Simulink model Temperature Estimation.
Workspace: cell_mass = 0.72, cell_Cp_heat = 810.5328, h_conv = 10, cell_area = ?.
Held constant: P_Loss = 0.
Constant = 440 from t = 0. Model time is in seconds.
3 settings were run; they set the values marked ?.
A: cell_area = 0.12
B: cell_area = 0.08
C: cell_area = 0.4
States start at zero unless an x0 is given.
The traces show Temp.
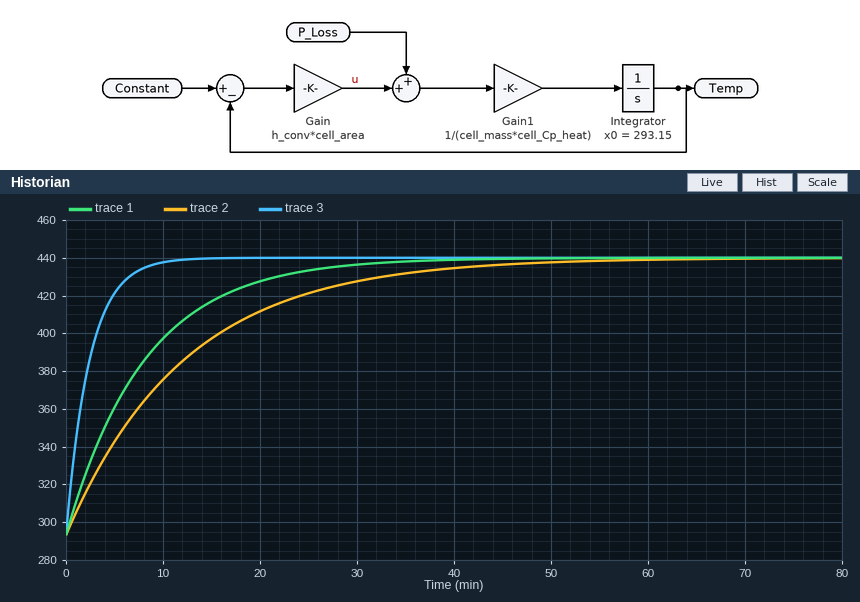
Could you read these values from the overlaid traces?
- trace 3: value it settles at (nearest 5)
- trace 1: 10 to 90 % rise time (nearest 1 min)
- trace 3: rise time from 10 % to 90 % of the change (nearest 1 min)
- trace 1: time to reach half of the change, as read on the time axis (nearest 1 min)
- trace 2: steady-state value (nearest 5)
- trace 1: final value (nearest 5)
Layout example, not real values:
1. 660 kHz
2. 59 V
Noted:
1. 440
2. 18 min
3. 5 min
4. 6 min
5. 440
6. 440
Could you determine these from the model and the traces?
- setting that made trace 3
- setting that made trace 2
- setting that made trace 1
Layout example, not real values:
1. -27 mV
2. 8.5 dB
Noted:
1. C
2. B
3. A
